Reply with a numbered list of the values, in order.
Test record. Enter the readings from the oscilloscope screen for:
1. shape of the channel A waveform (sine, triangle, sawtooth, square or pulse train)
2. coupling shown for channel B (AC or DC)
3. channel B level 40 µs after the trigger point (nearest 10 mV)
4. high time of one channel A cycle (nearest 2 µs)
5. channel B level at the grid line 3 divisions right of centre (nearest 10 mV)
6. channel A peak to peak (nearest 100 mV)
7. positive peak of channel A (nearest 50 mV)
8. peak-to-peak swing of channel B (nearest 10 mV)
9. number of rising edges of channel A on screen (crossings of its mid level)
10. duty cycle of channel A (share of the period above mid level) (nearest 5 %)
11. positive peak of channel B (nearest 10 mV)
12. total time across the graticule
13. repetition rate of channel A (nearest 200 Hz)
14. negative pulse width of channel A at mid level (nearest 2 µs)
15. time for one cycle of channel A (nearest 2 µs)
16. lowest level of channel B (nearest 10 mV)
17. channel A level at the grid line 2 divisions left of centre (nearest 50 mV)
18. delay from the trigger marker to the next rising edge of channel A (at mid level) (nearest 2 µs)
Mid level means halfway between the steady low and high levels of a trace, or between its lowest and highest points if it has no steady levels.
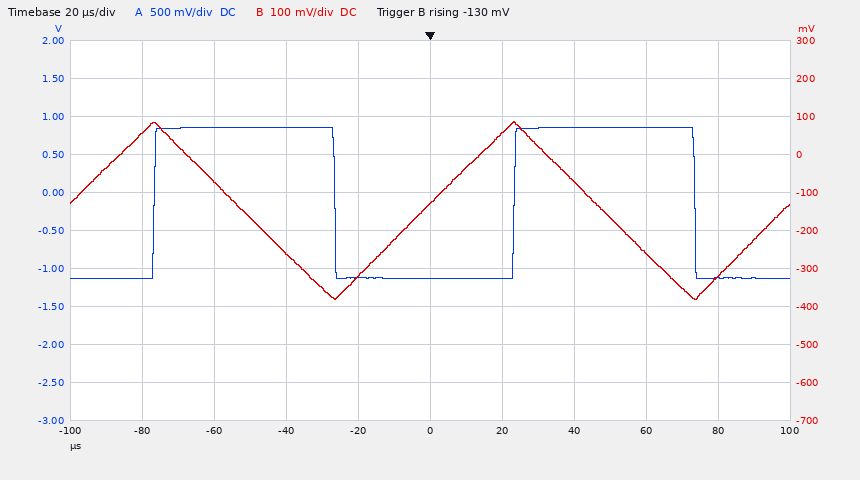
1. square
2. DC
3. -70 mV
4. 50 µs
5. -260 mV
6. 2.00 V
7. 850 mV
8. 470 mV
9. 2
10. 50 %
11. 90 mV
12. 200 µs
13. 10.0 kHz
14. 50 µs
15. 100 µs
16. -380 mV
17. 850 mV
18. 24 µs
